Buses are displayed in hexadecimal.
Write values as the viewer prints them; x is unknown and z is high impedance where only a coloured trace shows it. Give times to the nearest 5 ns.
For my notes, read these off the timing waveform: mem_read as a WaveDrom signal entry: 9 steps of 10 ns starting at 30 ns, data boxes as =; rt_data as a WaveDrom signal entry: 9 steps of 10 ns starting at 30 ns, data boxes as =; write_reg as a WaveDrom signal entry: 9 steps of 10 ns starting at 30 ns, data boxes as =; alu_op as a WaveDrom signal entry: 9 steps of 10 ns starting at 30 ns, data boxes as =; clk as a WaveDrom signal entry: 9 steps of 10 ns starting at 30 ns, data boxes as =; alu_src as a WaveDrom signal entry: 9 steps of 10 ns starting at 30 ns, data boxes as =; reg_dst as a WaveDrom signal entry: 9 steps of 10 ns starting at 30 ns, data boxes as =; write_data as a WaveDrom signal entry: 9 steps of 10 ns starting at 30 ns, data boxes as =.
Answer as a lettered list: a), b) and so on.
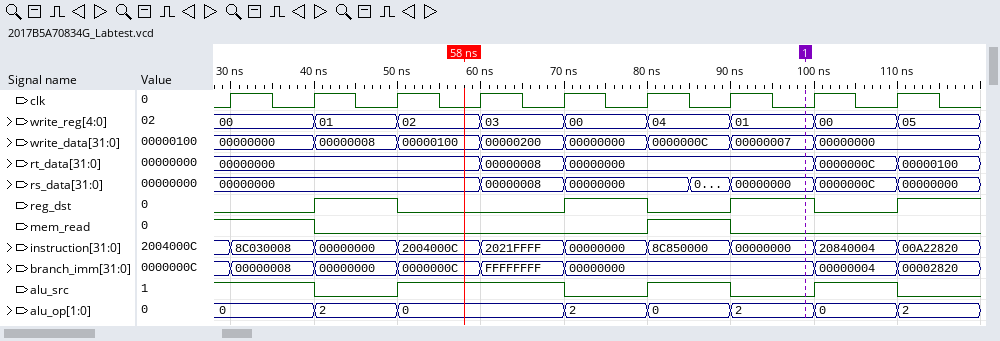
a) {name: 'mem_read', wave: '10...10..'}
b) {name: 'rt_data', wave: '=..==..==', data: '00000000 00000008 00000000 0000000C 00000100'}
c) {name: 'write_reg', wave: '=========', data: '00 01 02 03 00 04 01 00 05'}
d) {name: 'alu_op', wave: '===.=====', data: '0 2 0 2 0 2 0 2'}
e) {name: 'clk', wave: 'p........'}
f) {name: 'alu_src', wave: '101.01010'}
g) {name: 'reg_dst', wave: '010.10101'}
h) {name: 'write_data', wave: '========.', data: '00000000 00000008 00000100 00000200 00000000 0000000C 00000007 00000000'}
